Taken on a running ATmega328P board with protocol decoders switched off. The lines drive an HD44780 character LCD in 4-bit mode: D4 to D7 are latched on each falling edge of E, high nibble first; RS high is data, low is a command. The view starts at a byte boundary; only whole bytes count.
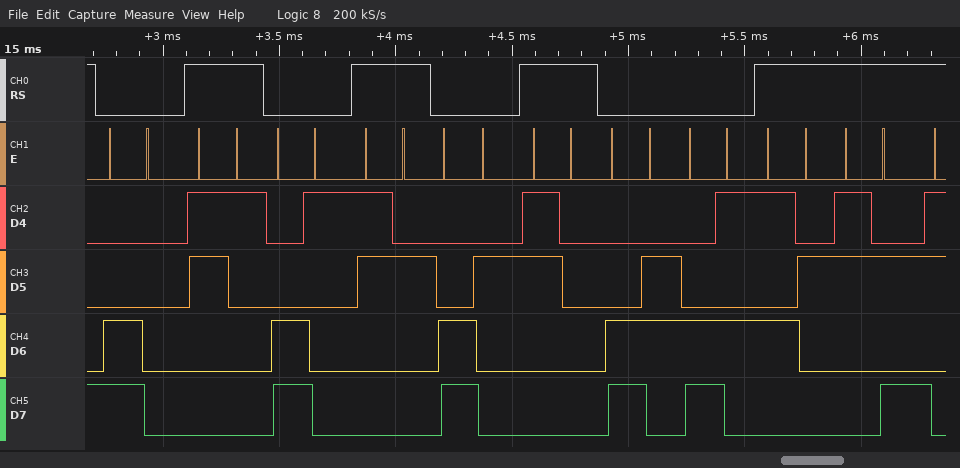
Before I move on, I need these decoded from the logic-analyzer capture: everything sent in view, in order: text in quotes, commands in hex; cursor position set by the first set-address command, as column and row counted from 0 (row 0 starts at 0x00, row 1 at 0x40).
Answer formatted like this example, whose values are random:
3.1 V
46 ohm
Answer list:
0xC0 "1" 0xC1 "2" 0xC2 "0" 0xC6 0xC5 "R:"
column 0, row 1
